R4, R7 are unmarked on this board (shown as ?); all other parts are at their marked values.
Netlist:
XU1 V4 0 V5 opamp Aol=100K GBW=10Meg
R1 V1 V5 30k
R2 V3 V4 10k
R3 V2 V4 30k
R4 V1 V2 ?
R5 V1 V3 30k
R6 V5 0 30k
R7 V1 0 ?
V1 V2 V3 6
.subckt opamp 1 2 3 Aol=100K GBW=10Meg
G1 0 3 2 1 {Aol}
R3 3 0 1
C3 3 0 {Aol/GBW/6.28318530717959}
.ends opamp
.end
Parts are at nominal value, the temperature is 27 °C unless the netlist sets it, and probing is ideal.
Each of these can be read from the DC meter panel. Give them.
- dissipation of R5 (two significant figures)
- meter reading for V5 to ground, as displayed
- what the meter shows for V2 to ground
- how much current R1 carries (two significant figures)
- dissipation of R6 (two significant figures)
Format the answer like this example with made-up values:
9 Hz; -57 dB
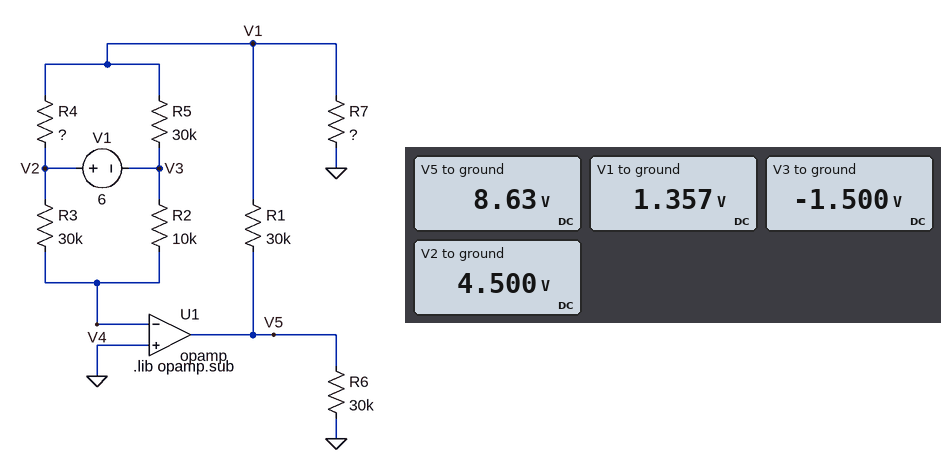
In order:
270 µW; 8.63 V; 4.500 V; 240 µA; 2.5 mW
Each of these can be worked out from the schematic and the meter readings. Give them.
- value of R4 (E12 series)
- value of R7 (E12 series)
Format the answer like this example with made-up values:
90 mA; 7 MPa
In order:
33 kΩ; 5.6 kΩ
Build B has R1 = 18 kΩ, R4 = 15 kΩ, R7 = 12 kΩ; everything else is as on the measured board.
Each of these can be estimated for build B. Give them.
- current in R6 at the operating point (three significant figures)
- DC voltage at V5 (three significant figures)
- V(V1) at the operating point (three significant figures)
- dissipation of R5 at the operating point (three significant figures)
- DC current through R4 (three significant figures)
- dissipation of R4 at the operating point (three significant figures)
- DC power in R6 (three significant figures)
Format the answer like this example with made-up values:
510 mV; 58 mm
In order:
208 µA; 6.25 V; 2.50 V; 533 µW; 133 µA; 267 µW; 1.30 mW
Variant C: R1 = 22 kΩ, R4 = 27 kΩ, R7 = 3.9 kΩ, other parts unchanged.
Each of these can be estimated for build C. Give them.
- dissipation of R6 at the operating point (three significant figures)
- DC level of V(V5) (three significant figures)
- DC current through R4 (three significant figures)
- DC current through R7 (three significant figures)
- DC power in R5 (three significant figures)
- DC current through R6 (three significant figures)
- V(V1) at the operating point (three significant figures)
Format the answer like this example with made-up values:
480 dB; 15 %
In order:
4.04 mW; 11.0 V; 105 µA; 425 µA; 332 µW; 367 µA; 1.66 V
